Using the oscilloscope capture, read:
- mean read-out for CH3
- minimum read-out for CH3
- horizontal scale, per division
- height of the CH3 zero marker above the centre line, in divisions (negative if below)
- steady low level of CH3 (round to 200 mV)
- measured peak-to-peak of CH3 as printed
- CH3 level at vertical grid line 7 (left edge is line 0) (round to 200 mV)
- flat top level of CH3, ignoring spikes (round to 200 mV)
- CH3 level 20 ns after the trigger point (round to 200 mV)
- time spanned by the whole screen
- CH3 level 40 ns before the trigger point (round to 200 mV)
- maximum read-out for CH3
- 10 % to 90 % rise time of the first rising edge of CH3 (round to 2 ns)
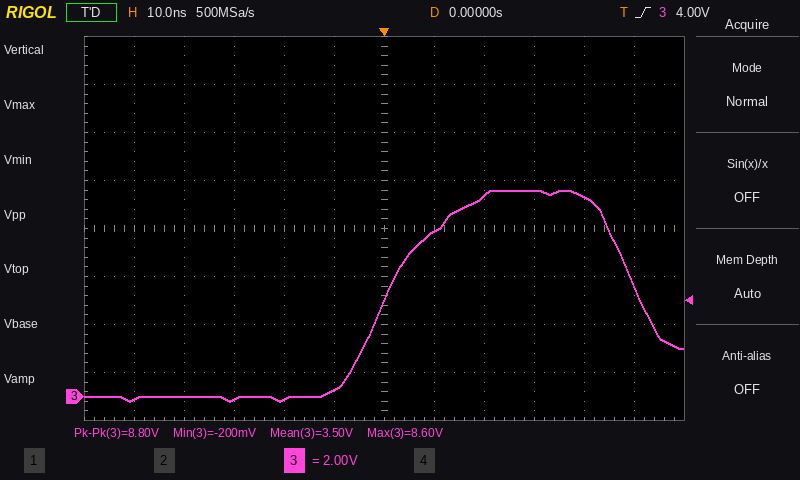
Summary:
3.50 V
-200 mV
10 ns
-3.5 div
0.0 V
8.80 V
6.8 V
8.6 V
8.4 V
120 ns
0.0 V
8.60 V
22 ns
